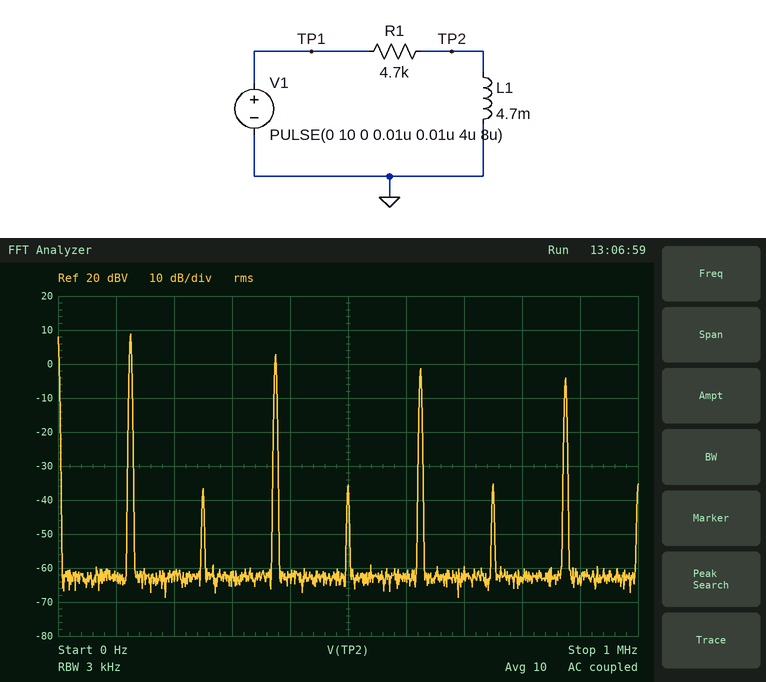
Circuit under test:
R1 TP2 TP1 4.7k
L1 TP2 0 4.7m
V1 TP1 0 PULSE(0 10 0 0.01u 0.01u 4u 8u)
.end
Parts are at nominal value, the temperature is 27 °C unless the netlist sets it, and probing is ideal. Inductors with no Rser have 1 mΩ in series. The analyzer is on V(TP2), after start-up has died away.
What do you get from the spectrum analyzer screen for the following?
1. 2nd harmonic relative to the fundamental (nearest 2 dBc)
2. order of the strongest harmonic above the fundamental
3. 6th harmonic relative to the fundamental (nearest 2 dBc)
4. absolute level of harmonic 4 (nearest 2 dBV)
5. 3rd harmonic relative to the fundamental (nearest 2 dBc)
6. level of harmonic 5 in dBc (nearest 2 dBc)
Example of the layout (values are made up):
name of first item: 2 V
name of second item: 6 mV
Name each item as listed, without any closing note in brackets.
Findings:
2nd harmonic relative to the fundamental: -46 dBc
order of the strongest harmonic above the fundamental: 3
6th harmonic relative to the fundamental: -44 dBc
absolute level of harmonic 4: -36 dBV
3rd harmonic relative to the fundamental: -6 dBc
level of harmonic 5 in dBc: -10 dBc
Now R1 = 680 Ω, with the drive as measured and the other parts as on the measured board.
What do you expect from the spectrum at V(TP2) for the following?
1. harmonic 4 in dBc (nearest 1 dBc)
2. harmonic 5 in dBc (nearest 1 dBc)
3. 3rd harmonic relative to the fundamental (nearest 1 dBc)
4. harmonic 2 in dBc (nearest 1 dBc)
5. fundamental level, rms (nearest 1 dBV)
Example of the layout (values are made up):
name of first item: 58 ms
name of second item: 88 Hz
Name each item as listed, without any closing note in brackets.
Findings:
harmonic 4 in dBc: -48 dBc
harmonic 5 in dBc: -14 dBc
3rd harmonic relative to the fundamental: -9 dBc
harmonic 2 in dBc: -48 dBc
fundamental level, rms: 13 dBV
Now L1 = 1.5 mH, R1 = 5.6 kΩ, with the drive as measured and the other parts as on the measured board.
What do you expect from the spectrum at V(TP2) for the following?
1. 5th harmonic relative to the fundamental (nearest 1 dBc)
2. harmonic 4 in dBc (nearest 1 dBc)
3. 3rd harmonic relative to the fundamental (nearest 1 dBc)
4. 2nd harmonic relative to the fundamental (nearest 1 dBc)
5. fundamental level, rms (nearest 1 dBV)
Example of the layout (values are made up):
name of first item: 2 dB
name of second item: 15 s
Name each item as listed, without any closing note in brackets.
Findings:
5th harmonic relative to the fundamental: -3 dBc
harmonic 4 in dBc: -38 dBc
3rd harmonic relative to the fundamental: -1 dBc
2nd harmonic relative to the fundamental: -43 dBc
fundamental level, rms: -1 dBV
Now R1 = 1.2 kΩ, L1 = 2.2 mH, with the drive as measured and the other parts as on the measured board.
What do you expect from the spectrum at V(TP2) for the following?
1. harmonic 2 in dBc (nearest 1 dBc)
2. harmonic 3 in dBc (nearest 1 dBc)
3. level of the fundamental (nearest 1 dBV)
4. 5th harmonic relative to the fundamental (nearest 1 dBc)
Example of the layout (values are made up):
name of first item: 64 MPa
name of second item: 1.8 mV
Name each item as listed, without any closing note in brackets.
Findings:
harmonic 2 in dBc: -47 dBc
harmonic 3 in dBc: -8 dBc
level of the fundamental: 11 dBV
5th harmonic relative to the fundamental: -12 dBc
